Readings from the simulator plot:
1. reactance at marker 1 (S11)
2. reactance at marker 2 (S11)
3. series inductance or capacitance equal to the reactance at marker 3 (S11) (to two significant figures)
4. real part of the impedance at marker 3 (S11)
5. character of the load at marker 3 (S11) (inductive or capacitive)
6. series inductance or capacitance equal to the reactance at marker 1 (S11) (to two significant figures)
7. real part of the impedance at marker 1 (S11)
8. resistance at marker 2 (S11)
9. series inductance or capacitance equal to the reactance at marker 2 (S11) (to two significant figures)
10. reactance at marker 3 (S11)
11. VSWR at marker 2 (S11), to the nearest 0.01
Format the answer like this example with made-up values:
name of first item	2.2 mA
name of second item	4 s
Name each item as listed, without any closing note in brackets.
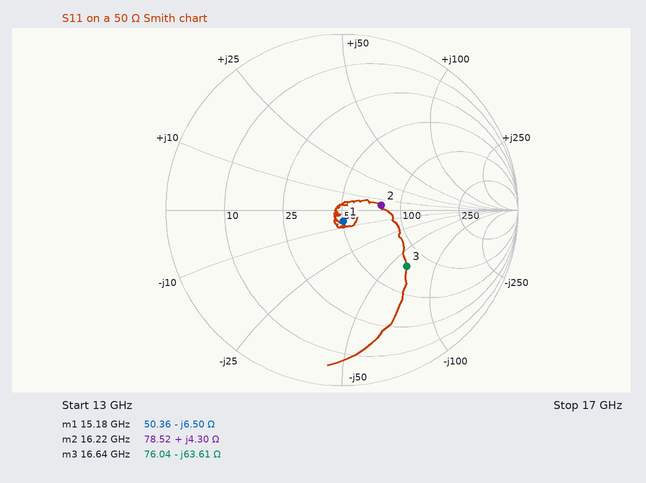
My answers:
reactance at marker 1	-6.50 Ω
reactance at marker 2	+4.30 Ω
series inductance or capacitance equal to the reactance at marker 3 (S11)	150 fF
real part of the impedance at marker 3	76.04 Ω
character of the load at marker 3 (S11)	capacitive
series inductance or capacitance equal to the reactance at marker 1 (S11)	1.6 pF
real part of the impedance at marker 1	50.36 Ω
resistance at marker 2	78.52 Ω
series inductance or capacitance equal to the reactance at marker 2 (S11)	42 pH
reactance at marker 3	-63.61 Ω
VSWR at marker 2 (S11), to the nearest 0.01	1.58
